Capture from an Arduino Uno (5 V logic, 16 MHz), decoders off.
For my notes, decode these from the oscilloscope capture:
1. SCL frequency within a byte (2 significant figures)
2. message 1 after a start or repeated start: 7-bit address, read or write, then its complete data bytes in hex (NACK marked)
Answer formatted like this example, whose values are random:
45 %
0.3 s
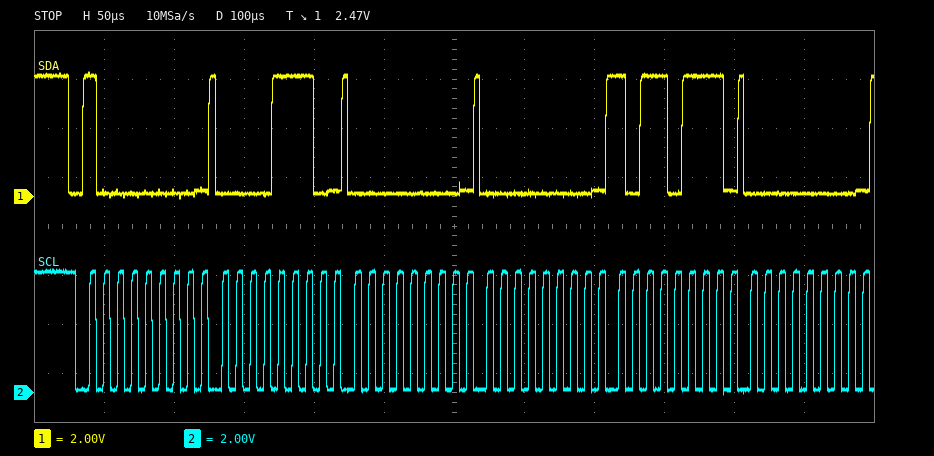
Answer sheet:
100 kHz
0x40 write: 0E 00 00 B7 00
